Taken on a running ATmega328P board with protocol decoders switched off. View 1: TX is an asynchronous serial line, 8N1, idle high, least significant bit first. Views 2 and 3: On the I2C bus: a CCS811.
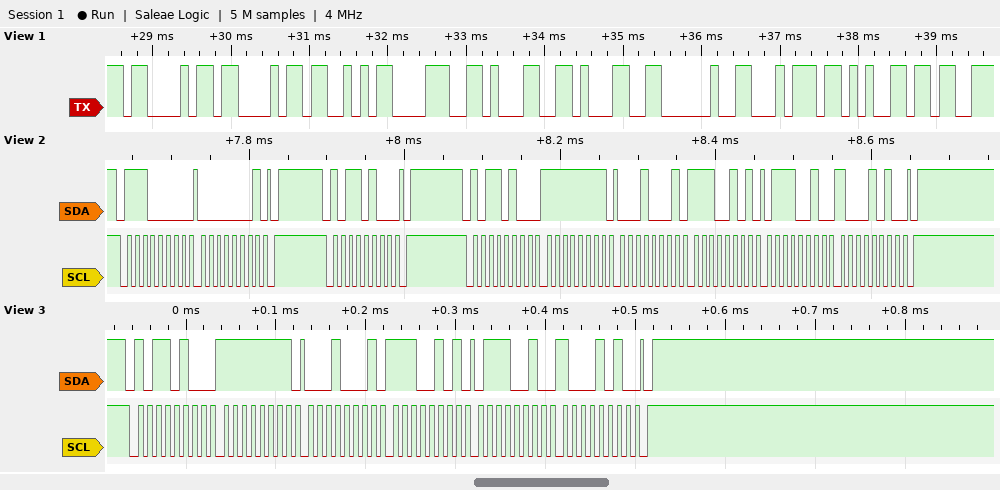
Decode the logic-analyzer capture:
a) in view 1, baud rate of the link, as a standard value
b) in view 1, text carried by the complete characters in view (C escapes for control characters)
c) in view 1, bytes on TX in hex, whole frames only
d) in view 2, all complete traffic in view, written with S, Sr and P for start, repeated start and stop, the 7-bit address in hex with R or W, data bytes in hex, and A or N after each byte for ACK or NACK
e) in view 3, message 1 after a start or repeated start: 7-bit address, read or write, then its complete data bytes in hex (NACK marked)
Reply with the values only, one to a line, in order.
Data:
9600 baud
"CCS811 te"
43 43 53 38 31 31 20 74 65
S 70W A 01 A P S 5AW A P S 5AW A FF A 11 A E5 A 72 A 8A A P
0x5A write: FF 11 E5 72 8A
